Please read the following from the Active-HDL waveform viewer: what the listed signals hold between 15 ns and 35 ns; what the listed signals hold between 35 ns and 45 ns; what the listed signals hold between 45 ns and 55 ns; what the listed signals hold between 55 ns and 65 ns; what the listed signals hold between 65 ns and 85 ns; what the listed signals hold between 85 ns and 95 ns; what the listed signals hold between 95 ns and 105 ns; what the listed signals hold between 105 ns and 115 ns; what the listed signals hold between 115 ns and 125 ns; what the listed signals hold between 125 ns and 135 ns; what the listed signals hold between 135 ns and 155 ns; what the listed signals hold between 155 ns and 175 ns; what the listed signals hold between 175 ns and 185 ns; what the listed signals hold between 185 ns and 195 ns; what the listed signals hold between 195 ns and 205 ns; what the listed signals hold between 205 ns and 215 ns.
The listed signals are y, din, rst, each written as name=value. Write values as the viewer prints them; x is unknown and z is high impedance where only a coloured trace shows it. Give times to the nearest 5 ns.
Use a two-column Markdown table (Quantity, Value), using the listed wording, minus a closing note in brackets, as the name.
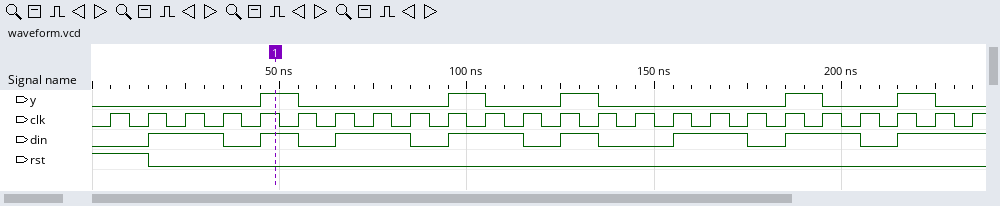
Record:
| Quantity | Value |
|---|---|
| what the listed signals hold between 15 ns and 35 ns | y=0, din=1, rst=0 |
| what the listed signals hold between 35 ns and 45 ns | y=0, din=0, rst=0 |
| what the listed signals hold between 45 ns and 55 ns | y=1, din=1, rst=0 |
| what the listed signals hold between 55 ns and 65 ns | y=0, din=0, rst=0 |
| what the listed signals hold between 65 ns and 85 ns | y=0, din=1, rst=0 |
| what the listed signals hold between 85 ns and 95 ns | y=0, din=0, rst=0 |
| what the listed signals hold between 95 ns and 105 ns | y=1, din=1, rst=0 |
| what the listed signals hold between 105 ns and 115 ns | y=0, din=1, rst=0 |
| what the listed signals hold between 115 ns and 125 ns | y=0, din=0, rst=0 |
| what the listed signals hold between 125 ns and 135 ns | y=1, din=1, rst=0 |
| what the listed signals hold between 135 ns and 155 ns | y=0, din=0, rst=0 |
| what the listed signals hold between 155 ns and 175 ns | y=0, din=1, rst=0 |
| what the listed signals hold between 175 ns and 185 ns | y=0, din=0, rst=0 |
| what the listed signals hold between 185 ns and 195 ns | y=1, din=1, rst=0 |
| what the listed signals hold between 195 ns and 205 ns | y=0, din=1, rst=0 |
| what the listed signals hold between 205 ns and 215 ns | y=0, din=0, rst=0 |
